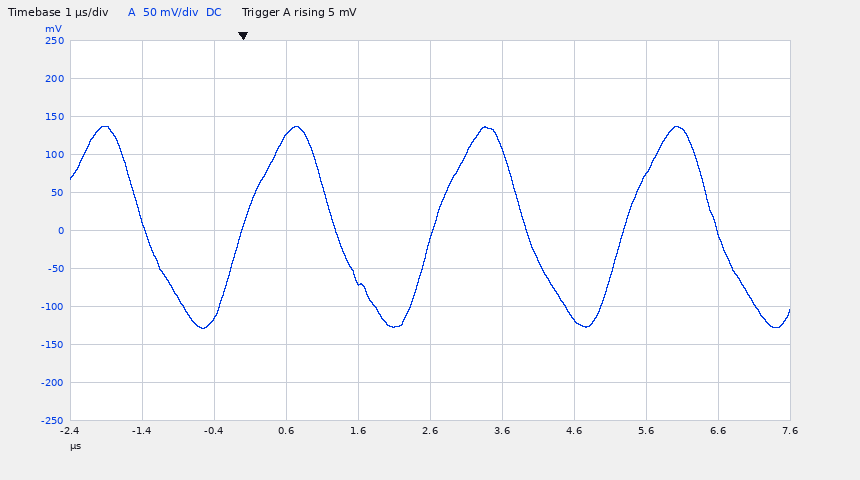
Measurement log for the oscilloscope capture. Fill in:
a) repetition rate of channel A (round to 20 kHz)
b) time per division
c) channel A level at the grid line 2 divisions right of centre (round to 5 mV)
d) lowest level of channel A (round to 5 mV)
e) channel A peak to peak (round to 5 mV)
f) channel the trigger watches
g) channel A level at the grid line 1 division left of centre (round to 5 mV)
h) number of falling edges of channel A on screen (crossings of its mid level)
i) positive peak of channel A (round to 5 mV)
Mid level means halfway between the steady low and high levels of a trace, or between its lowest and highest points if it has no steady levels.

380 kHz
1 µs
-115 mV
-130 mV
265 mV
channel A
-65 mV
4
135 mV
